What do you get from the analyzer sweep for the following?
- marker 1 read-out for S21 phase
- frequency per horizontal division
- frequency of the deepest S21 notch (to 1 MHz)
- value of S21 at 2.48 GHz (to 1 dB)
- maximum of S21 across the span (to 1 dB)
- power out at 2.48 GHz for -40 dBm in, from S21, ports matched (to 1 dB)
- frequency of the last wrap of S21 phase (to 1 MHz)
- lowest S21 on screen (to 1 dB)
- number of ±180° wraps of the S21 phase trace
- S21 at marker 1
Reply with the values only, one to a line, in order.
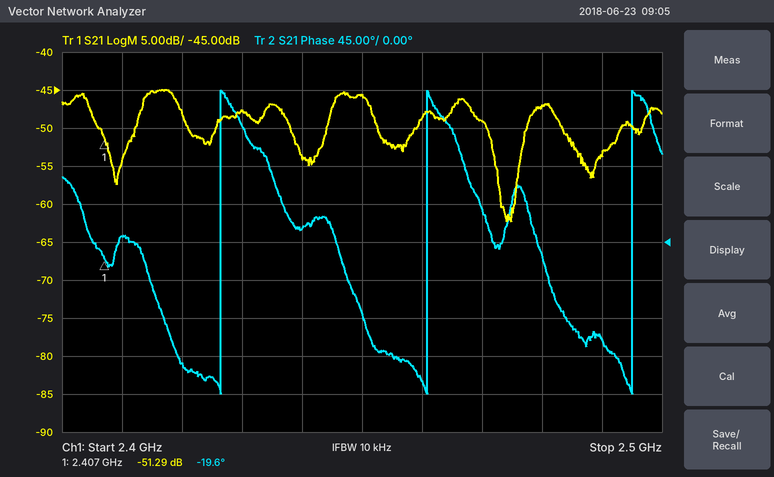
-19.6°
10 MHz
2.474 GHz
-47 dB
-45 dB
-87 dBm
2.495 GHz
-62 dB
3
-51.29 dB
